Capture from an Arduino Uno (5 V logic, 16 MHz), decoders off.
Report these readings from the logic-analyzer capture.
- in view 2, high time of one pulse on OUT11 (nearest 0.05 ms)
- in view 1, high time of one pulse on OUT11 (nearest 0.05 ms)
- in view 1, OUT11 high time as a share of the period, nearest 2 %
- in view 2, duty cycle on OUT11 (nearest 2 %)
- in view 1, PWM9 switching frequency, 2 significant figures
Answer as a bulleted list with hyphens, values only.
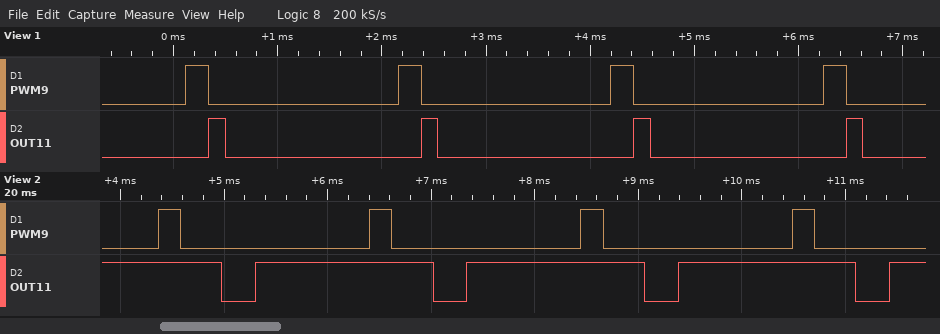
- 1.70 ms
- 0.15 ms
- 8 %
- 84 %
- 490 Hz
